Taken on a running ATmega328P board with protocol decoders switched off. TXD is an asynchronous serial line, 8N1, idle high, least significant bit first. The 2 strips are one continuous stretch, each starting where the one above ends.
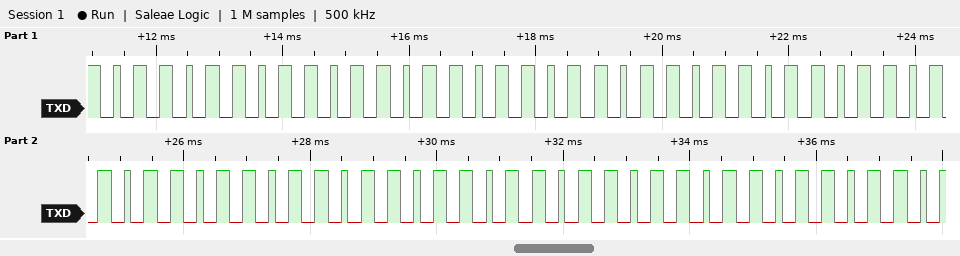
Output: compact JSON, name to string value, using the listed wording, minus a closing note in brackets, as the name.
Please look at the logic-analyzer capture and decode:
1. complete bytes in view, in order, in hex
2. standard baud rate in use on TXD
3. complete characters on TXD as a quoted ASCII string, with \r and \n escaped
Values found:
{"complete bytes in view, in order, in hex": "32 32 32 32 32 32 32 32 32 32 32 32 32 32 32 32 32 32 32 32 32 32 32", "standard baud rate in use on TXD": "9600 baud", "complete characters on TXD as a quoted ASCII string, with \\r and \\n escaped": "\"22222222222222222222222\""}
